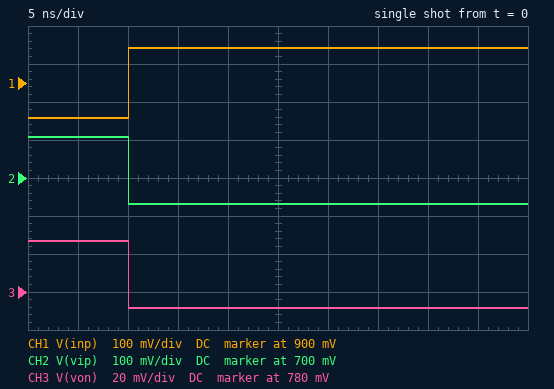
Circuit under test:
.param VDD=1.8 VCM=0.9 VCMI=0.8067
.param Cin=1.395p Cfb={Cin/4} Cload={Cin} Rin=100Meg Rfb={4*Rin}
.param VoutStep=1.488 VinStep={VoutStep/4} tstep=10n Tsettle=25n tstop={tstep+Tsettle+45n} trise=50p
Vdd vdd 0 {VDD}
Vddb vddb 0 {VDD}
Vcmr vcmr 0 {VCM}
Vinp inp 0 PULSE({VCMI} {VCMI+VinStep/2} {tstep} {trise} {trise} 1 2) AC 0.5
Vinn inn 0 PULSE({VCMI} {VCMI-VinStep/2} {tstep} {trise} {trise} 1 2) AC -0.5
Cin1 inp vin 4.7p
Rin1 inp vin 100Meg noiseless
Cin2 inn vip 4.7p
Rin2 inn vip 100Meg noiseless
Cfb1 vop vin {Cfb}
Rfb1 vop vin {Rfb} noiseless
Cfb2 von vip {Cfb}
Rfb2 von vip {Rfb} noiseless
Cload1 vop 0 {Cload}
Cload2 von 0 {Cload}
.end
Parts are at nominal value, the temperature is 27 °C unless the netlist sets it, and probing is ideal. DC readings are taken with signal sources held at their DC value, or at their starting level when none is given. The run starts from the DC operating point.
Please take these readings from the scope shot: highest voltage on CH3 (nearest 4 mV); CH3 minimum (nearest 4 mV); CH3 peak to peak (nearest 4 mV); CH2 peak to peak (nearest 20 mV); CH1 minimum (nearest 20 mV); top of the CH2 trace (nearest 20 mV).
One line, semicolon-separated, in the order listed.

808 mV; 772 mV; 36 mV; 180 mV; 800 mV; 800 mV
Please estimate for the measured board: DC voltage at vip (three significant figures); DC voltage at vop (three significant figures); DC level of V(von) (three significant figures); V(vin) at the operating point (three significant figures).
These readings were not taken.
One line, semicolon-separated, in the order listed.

807 mV; 807 mV; 807 mV; 807 mV
